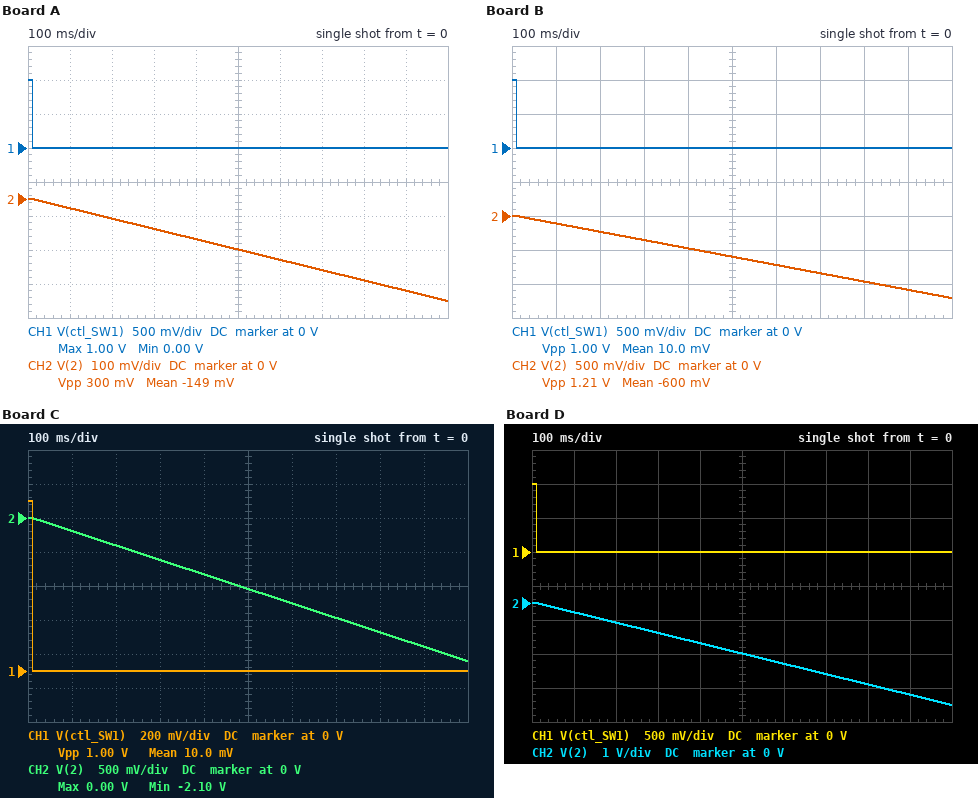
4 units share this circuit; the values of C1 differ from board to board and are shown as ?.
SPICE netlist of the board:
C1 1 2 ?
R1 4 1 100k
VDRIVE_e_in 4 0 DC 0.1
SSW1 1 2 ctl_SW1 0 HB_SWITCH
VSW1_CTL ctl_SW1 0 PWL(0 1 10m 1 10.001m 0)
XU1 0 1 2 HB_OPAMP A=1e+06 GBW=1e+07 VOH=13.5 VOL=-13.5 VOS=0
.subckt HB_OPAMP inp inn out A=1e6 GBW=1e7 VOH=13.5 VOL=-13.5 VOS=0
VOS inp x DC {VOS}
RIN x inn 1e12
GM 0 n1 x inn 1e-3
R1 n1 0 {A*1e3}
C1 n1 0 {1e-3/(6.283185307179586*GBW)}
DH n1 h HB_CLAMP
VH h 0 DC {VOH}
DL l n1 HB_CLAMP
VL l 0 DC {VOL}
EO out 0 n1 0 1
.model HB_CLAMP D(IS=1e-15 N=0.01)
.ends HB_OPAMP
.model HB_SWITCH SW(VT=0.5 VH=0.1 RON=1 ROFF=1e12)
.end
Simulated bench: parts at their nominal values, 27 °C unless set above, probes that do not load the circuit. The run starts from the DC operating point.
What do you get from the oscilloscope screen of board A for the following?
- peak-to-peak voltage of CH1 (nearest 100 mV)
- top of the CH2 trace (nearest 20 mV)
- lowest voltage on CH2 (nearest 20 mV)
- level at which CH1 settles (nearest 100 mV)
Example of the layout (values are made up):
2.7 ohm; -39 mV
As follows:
1.0 V; 0 V; -300 mV; 0 V
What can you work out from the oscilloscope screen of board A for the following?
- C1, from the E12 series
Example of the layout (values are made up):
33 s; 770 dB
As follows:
3.3 µF
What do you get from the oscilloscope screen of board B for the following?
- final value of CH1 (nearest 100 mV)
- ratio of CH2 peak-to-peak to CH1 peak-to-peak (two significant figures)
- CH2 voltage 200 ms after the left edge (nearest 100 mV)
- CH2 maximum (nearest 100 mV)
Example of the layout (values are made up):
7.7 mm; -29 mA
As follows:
0 V; 1.2; -200 mV; 0 V
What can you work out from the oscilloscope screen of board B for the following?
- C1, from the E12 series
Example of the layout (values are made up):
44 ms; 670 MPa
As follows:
820 nF
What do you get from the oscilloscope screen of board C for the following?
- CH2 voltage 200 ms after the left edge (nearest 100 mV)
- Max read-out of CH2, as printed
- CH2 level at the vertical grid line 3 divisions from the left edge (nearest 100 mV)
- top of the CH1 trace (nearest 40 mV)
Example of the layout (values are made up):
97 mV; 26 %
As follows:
-400 mV; 0.00 V; -600 mV; 1.00 V
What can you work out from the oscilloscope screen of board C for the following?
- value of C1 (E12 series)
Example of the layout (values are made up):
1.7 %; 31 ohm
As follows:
470 nF
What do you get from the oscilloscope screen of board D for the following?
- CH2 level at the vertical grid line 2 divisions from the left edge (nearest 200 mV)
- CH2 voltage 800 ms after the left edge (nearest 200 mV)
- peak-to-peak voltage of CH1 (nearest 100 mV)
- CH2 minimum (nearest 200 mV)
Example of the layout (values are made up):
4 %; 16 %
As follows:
-600 mV; -2.4 V; 1.0 V; -3.0 V
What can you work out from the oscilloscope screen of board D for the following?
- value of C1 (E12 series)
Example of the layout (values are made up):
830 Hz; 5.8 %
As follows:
330 nF
